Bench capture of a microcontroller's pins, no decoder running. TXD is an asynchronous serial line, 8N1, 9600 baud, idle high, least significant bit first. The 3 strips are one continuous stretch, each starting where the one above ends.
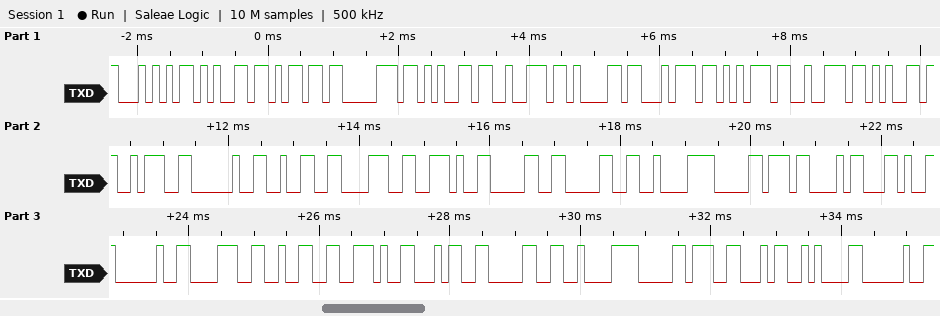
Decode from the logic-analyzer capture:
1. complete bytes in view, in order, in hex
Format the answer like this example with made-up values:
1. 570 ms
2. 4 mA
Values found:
1. 0x54 0x65 0x6D 0x70 0x65 0x72 0x61 0x74 0x75 0x72 0x65 0x3A 0x20 0x32 0x38 0x2E 0x30 0x30 0xC2 0xB0 0x43 0x2C 0x20 0x38 0x32 0x2E 0x34 0x30 0xC2 0xB0 0x46 0x0A 0x20
